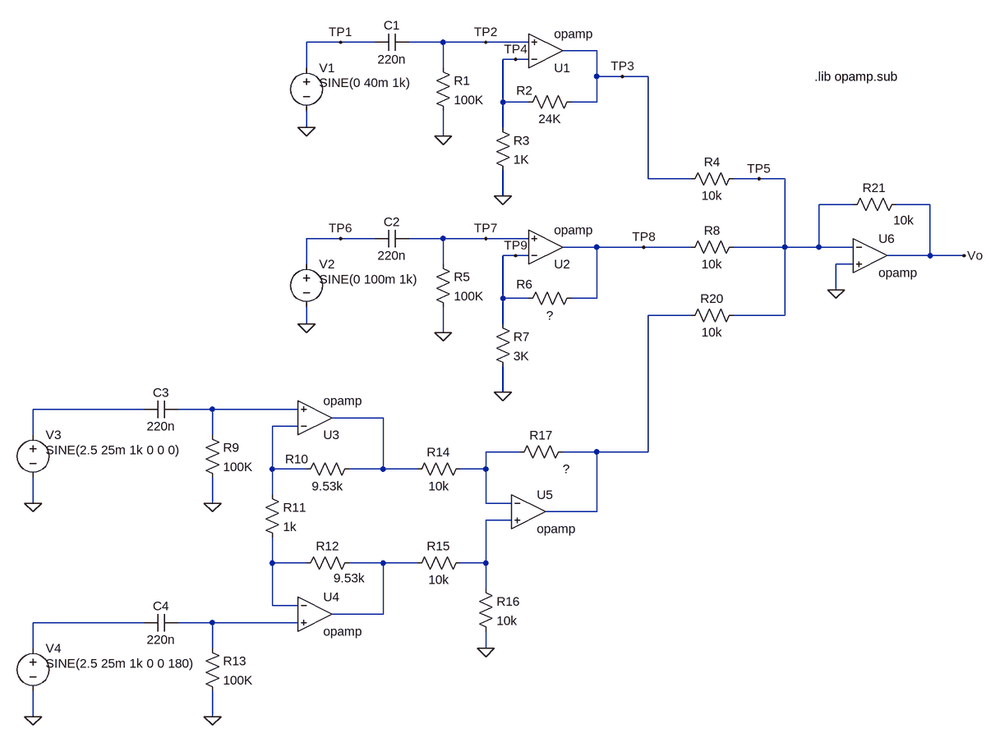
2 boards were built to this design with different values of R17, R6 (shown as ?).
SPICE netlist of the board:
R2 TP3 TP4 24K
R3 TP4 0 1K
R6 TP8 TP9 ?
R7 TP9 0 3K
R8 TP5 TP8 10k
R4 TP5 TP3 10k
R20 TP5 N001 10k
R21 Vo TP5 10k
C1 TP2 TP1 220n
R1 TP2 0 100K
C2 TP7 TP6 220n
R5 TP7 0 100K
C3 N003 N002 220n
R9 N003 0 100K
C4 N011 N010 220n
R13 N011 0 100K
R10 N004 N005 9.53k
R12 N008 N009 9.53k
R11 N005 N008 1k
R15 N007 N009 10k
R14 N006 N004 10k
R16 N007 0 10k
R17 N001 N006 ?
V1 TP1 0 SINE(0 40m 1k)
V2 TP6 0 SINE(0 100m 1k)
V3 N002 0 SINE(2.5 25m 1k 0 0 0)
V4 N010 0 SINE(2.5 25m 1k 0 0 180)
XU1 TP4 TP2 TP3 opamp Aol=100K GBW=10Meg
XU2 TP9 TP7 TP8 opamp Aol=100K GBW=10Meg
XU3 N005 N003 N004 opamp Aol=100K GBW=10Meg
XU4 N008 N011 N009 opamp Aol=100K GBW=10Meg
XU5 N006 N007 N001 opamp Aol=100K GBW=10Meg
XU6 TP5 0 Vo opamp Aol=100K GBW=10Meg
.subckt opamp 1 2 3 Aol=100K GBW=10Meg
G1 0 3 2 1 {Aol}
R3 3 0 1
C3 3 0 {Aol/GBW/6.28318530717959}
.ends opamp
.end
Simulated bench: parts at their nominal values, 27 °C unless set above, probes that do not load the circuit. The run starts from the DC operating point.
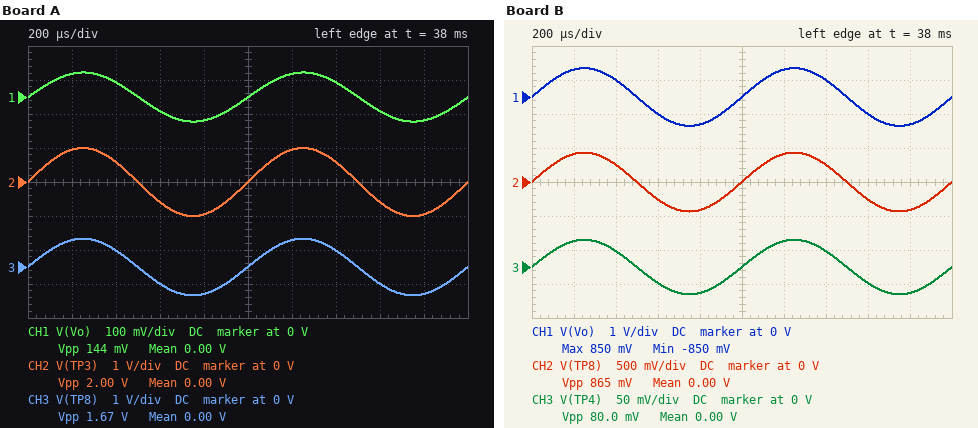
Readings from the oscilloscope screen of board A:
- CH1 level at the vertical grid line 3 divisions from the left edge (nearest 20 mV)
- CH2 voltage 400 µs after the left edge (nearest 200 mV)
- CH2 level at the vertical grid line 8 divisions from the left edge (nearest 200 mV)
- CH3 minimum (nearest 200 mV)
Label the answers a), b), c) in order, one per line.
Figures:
a) -40 mV
b) 600 mV
c) -600 mV
d) -800 mV
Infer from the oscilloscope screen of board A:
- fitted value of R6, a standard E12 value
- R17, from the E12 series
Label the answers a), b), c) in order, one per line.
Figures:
a) 22 kΩ
b) 22 kΩ
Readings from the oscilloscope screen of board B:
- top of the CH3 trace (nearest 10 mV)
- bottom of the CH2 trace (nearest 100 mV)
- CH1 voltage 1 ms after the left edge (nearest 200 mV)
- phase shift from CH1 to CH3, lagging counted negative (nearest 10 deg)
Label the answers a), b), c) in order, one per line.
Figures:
a) 40 mV
b) -400 mV
c) 0 V
d) 0 deg
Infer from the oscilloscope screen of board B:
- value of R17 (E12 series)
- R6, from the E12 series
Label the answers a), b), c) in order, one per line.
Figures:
a) 27 kΩ
b) 10 kΩ
